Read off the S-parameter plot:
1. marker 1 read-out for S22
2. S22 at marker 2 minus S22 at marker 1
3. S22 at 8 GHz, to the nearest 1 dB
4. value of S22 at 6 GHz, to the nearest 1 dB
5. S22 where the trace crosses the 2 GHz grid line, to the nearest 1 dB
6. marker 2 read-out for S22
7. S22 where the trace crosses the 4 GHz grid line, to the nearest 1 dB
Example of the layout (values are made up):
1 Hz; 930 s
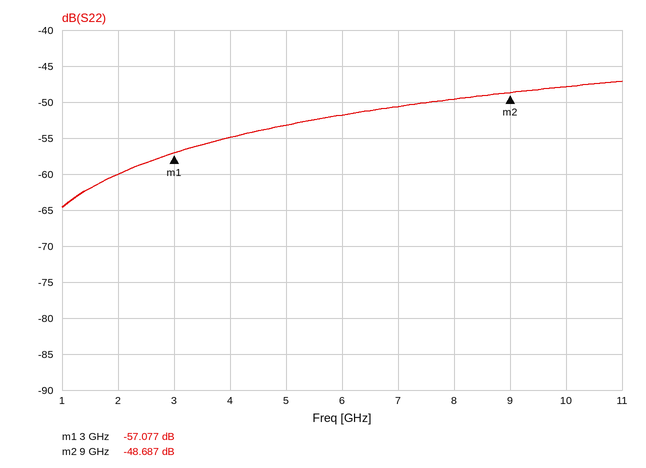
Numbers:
-57.077 dB; 8.390 dB; -50 dB; -52 dB; -60 dB; -48.687 dB; -55 dB
